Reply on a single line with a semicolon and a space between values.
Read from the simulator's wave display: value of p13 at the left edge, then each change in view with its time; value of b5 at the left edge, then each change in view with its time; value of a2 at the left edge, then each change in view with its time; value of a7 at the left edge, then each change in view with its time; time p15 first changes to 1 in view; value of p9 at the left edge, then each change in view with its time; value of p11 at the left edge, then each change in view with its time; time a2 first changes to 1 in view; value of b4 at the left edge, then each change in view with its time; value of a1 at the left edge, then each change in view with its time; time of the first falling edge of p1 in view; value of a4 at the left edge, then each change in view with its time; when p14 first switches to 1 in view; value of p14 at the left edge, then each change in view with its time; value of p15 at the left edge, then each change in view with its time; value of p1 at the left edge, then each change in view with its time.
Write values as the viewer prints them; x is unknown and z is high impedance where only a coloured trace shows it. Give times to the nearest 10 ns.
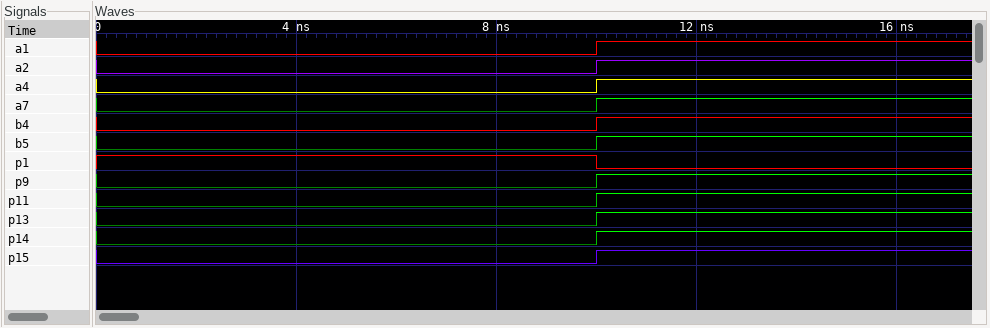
0, 1 at 10 ns; 0, 1 at 10 ns; 0, 1 at 10 ns; 0, 1 at 10 ns; 10 ns; 0, 1 at 10 ns; 0, 1 at 10 ns; 10 ns; 0, 1 at 10 ns; 0, 1 at 10 ns; 10 ns; 0, 1 at 10 ns; 10 ns; 0, 1 at 10 ns; 0, 1 at 10 ns; 1, 0 at 10 ns
